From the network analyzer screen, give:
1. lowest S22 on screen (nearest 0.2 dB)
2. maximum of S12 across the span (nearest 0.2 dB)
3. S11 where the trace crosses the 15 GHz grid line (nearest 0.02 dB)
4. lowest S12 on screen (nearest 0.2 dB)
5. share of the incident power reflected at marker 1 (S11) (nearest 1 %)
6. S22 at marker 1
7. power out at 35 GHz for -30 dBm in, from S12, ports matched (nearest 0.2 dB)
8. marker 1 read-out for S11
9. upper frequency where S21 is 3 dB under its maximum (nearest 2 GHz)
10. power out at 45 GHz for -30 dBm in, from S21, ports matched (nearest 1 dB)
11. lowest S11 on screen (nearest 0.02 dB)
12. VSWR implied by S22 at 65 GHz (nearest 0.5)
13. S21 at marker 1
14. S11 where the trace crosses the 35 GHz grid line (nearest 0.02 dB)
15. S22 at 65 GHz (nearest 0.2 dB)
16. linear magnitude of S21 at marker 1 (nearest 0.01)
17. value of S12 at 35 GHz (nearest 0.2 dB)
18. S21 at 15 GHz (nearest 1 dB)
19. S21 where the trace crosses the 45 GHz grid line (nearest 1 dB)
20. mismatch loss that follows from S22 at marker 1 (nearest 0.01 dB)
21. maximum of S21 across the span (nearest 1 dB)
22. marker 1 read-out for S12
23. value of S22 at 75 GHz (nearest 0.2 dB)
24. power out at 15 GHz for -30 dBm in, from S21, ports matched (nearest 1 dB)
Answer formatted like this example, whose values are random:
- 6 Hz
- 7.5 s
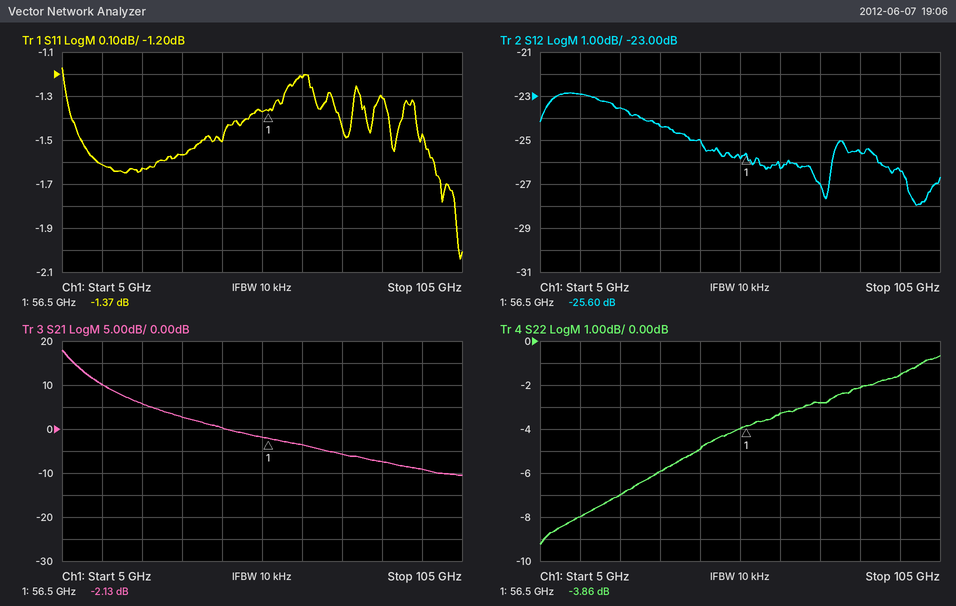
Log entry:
- -9.2 dB
- -22.8 dB
- -1.62 dB
- -28.0 dB
- 73 %
- -3.86 dB
- -54.4 dBm
- -1.37 dB
- 8 GHz
- -30 dBm
- -2.04 dB
- 5.5
- -2.13 dB
- -1.56 dB
- -3.2 dB
- 0.78
- -24.4 dB
- 10 dB
- 0 dB
- 2.30 dB
- 18 dB
- -25.60 dB
- -2.8 dB
- -20 dBm
